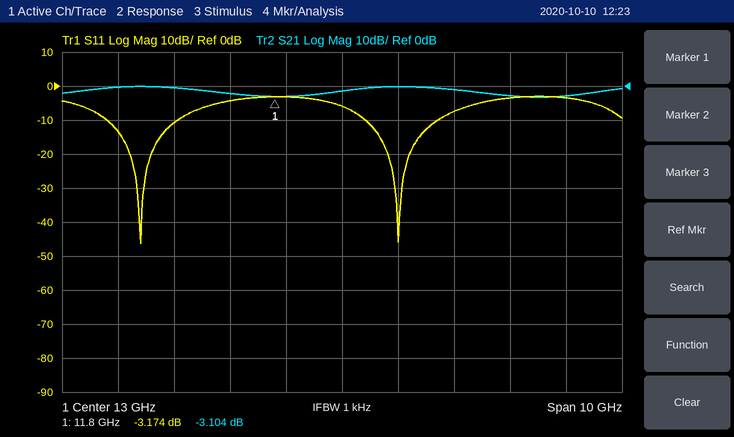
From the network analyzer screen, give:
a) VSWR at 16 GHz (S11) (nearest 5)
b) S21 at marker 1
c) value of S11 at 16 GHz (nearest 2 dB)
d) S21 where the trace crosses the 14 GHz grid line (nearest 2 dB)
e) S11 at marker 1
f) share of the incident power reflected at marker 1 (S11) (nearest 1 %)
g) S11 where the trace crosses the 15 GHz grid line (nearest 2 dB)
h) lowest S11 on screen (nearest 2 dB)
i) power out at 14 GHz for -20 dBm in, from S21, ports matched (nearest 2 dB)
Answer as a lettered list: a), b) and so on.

a) 5
b) -3.104 dB
c) -4 dB
d) 0 dB
e) -3.174 dB
f) 48 %
g) -8 dB
h) -46 dB
i) -20 dBm
